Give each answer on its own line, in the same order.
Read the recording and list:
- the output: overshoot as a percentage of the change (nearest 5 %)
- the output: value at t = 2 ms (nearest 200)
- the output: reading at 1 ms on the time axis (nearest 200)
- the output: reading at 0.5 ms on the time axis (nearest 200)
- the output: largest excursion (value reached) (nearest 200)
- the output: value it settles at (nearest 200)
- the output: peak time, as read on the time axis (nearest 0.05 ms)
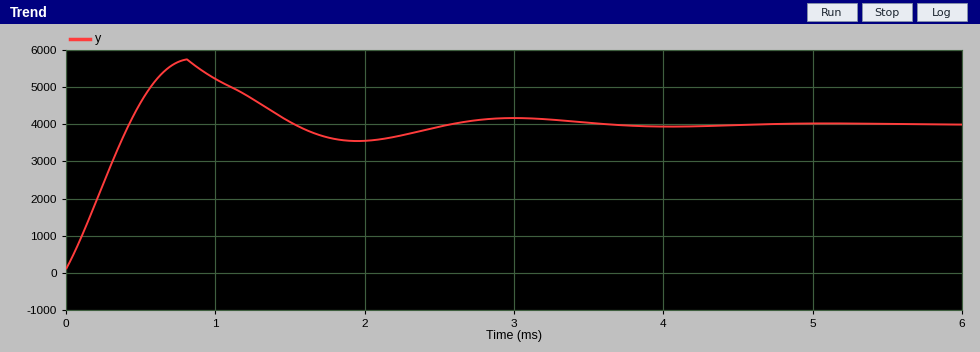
45 %
3600
5200
4600
5800
4000
0.80 ms
